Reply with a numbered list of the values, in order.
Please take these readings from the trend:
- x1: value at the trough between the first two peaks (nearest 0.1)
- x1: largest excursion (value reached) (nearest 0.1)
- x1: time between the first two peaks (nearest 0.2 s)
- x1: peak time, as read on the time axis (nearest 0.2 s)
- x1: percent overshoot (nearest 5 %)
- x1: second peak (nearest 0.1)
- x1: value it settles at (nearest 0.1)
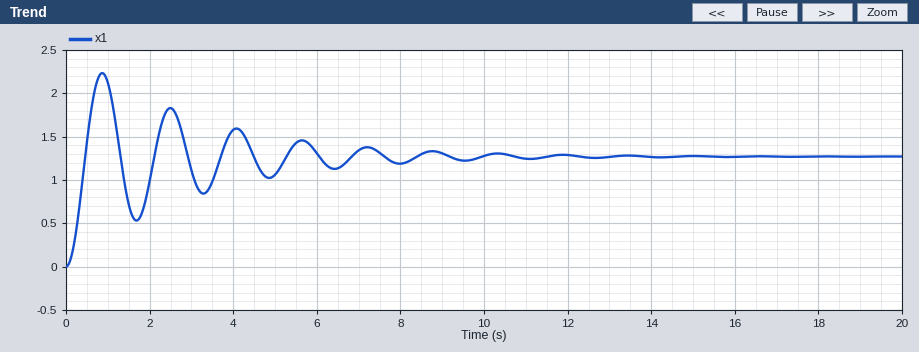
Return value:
1. 0.5
2. 2.2
3. 1.6 s
4. 0.8 s
5. 75 %
6. 1.8
7. 1.3
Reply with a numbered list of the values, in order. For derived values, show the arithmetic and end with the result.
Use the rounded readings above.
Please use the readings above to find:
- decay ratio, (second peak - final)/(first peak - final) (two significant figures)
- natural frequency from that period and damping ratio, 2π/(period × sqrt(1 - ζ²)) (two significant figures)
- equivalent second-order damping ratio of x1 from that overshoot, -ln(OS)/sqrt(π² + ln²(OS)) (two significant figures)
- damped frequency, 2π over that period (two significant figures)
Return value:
1. (1.8 - 1.3) / (2.2 - 1.3) = 0.56
2. 2π / (1.6 × sqrt(1 - 0.091²)) = 3.9 rad/s
3. ln(0.75) = -0.288; 0.288 / sqrt(9.870 + 0.083) = 0.091
4. 2π / 1.6 = 3.9 rad/s
